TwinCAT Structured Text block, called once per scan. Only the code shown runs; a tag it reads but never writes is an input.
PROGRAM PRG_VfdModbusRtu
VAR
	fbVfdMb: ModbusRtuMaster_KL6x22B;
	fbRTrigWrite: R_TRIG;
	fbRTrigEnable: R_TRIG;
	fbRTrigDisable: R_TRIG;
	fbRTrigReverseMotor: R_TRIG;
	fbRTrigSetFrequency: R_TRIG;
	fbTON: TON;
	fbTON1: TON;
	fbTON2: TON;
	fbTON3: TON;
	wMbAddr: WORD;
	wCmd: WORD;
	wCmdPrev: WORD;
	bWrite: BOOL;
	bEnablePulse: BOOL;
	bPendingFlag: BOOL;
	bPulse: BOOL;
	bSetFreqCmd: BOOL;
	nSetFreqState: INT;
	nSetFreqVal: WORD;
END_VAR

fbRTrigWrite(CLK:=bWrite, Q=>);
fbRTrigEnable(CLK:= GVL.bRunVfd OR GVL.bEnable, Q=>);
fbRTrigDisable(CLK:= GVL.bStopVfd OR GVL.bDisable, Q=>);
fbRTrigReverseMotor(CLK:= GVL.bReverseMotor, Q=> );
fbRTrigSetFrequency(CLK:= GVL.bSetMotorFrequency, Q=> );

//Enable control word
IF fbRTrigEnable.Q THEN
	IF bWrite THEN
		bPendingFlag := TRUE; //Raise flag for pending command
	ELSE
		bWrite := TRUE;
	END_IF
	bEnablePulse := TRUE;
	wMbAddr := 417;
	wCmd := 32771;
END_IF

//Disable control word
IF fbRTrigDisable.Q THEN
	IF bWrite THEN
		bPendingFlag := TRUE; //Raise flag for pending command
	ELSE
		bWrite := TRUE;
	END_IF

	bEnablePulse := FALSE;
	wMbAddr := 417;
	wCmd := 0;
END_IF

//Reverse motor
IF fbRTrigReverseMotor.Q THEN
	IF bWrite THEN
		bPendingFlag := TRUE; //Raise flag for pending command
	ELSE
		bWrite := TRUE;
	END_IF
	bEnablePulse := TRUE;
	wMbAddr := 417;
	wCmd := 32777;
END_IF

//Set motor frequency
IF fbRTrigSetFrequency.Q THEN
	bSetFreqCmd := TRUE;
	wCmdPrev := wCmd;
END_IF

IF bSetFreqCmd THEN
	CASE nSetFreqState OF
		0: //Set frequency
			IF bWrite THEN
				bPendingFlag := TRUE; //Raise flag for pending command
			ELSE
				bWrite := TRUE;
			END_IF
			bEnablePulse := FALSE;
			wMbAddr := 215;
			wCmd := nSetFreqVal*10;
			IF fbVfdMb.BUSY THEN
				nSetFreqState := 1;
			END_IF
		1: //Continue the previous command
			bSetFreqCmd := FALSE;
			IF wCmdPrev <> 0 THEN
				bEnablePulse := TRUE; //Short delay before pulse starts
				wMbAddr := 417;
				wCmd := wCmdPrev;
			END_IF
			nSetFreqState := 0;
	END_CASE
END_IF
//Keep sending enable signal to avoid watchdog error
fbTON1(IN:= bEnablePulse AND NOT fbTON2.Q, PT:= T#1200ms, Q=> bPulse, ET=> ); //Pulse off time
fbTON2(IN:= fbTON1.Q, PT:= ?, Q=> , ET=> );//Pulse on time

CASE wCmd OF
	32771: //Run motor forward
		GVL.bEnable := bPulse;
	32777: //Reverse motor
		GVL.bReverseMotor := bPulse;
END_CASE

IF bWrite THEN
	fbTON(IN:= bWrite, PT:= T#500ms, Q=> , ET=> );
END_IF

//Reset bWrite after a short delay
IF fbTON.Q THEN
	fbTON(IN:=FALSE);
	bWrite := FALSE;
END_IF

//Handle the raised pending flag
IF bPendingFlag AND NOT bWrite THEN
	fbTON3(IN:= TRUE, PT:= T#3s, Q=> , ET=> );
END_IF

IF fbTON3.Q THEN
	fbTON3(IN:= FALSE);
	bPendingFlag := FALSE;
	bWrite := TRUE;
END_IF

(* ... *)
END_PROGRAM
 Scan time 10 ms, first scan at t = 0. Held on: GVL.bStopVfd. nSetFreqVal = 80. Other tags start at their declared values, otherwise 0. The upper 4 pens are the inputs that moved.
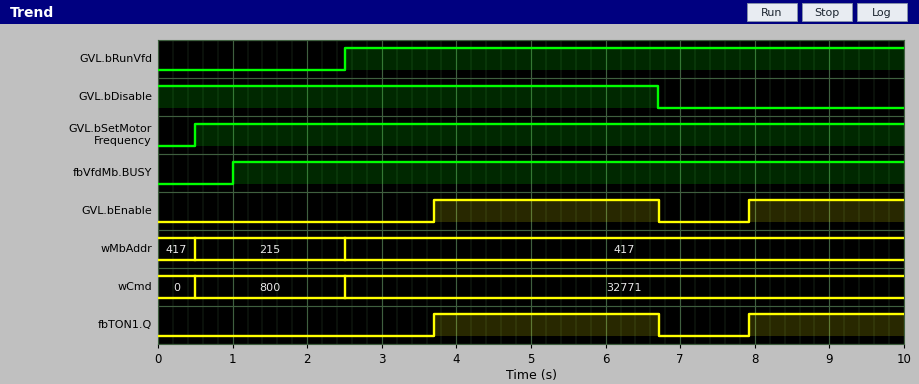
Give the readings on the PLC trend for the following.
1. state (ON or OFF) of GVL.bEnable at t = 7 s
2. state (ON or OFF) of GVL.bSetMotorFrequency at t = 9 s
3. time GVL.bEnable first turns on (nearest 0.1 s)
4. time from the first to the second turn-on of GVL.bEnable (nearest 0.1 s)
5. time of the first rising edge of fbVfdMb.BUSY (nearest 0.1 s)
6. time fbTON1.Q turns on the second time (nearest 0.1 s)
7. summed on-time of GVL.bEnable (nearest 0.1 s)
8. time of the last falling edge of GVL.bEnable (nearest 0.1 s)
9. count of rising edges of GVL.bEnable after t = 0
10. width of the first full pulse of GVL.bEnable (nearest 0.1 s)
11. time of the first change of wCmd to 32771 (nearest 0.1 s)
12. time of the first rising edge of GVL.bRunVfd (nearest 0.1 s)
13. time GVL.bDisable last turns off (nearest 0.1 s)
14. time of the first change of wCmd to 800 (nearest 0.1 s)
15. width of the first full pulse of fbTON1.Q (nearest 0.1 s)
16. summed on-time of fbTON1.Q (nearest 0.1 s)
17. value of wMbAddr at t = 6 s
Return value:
OFF
ON
3.7 s
4.2 s
1.0 s
7.9 s
5.1 s
6.7 s
2
3.0 s
2.5 s
2.5 s
6.7 s
0.5 s
3.0 s
5.1 s
417
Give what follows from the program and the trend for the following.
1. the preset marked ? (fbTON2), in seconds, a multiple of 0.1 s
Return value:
3.0 s
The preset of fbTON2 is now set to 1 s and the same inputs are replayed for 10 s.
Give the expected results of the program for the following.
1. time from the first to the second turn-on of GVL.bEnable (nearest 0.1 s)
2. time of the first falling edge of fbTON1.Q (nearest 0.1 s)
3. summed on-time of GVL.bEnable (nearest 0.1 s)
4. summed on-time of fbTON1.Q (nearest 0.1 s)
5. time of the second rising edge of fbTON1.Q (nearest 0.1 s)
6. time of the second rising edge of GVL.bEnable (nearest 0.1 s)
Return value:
2.2 s
4.7 s
3.0 s
3.0 s
5.9 s
5.9 s
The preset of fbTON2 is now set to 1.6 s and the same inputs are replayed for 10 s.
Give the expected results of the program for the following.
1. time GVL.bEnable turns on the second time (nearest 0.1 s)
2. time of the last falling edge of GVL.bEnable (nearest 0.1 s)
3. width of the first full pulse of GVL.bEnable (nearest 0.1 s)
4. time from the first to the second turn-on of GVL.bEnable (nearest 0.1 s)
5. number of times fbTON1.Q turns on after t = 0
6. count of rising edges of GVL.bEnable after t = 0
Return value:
6.5 s
8.1 s
1.6 s
2.8 s
3
3
